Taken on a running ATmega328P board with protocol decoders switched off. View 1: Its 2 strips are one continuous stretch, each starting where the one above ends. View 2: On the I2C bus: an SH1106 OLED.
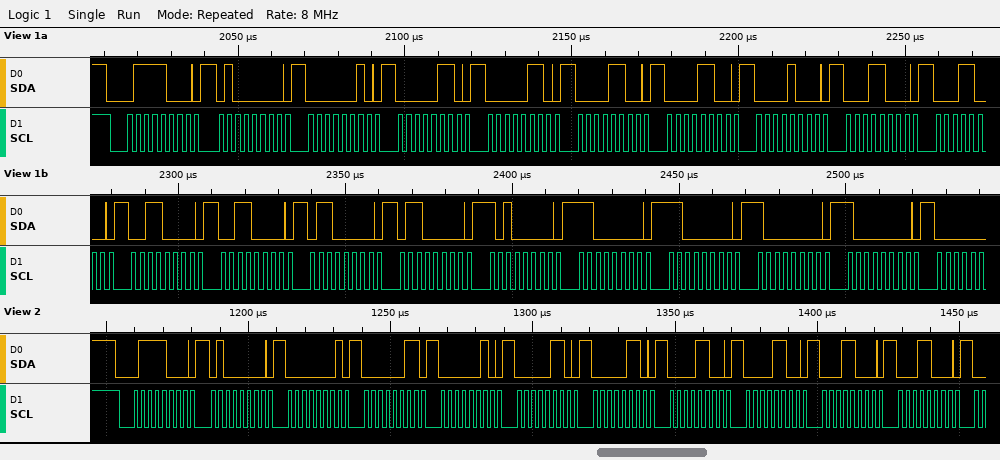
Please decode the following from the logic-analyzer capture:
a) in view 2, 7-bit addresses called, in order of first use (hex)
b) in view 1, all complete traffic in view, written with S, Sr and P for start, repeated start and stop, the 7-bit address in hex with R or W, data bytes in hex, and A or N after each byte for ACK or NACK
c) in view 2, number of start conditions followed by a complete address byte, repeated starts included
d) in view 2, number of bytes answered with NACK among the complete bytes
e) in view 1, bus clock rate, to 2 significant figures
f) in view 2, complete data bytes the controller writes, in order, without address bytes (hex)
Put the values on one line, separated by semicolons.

0x3C; S 3CW A 40 A 02 A 06 A 06 A 0C A 0C A 08 A 18 A 18 A 30 A 30 A 60 A 60 A A0 A C0 A C0 A 80 A 80 A; 1; 0; 400 kHz; 40 01 03 02 06 06 0C 0C 18 18
